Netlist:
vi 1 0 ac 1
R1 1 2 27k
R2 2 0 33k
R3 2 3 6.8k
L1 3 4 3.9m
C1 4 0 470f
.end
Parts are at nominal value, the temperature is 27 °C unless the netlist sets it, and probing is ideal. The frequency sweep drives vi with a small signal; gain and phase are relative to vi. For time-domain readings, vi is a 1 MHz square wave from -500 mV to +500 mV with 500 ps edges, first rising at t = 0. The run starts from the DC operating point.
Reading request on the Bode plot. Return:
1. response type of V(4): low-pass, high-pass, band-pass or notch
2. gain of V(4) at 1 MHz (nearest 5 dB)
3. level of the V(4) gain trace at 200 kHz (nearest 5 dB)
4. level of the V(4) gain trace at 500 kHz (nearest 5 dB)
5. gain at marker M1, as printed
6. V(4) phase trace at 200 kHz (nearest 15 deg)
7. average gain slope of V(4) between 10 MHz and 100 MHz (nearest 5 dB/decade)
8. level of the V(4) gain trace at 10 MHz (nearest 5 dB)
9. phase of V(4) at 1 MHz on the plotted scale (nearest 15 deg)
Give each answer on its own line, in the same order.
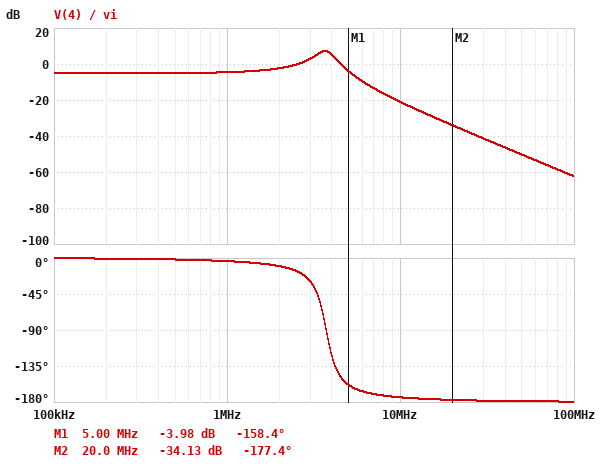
low-pass
-5 dB
-5 dB
-5 dB
-3.98 dB
0 deg
-40 dB/decade
-20 dB
0 deg
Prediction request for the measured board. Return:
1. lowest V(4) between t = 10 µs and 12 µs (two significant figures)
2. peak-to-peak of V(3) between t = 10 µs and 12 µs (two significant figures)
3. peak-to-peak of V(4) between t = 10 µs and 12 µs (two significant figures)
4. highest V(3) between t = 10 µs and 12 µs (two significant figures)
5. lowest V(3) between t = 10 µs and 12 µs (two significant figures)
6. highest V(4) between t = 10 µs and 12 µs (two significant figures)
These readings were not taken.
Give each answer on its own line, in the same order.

-610 mV
680 mV
1.2 V
340 mV
-340 mV
610 mV
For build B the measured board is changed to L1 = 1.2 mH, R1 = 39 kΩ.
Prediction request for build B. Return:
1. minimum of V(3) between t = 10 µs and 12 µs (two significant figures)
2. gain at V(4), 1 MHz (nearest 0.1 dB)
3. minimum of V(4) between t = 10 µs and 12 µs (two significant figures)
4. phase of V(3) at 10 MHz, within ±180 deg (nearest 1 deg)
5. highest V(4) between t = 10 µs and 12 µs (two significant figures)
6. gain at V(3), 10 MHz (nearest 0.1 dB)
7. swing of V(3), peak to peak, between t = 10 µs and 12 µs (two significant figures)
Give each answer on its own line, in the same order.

-300 mV
-6.6 dB
-440 mV
31 deg
440 mV
-8.1 dB
600 mV
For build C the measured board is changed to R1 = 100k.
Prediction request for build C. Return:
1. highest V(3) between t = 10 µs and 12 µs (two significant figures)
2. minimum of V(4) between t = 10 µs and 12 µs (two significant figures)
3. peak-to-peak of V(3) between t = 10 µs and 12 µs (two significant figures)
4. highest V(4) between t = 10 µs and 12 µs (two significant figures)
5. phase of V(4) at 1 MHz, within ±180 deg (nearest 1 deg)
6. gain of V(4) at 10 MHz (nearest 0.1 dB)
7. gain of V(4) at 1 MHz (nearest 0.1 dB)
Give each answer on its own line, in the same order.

160 mV
-260 mV
320 mV
260 mV
-6 deg
-28.1 dB
-11.5 dB
